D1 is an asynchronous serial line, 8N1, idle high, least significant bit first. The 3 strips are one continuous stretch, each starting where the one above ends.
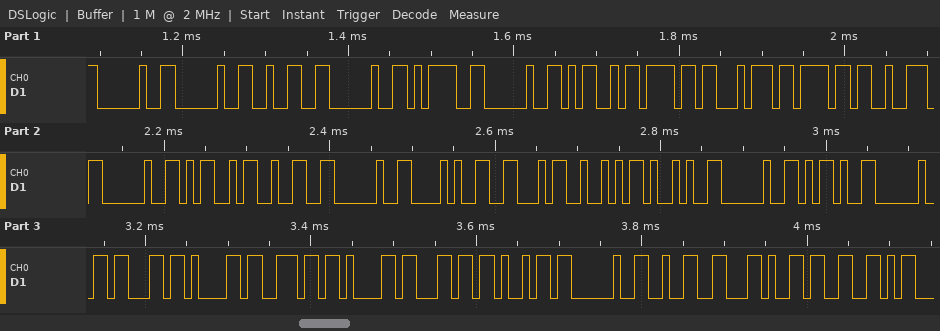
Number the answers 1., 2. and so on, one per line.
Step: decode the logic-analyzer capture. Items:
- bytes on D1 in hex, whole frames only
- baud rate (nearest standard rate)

1. 20 20 32 20 3D 20 4D 6F 74 6F 72 20 4D 32 20 28 46 52 29 20 2D 20 63 61 6E 61 6C 69 20 32 2C 33
2. 115200 baud
